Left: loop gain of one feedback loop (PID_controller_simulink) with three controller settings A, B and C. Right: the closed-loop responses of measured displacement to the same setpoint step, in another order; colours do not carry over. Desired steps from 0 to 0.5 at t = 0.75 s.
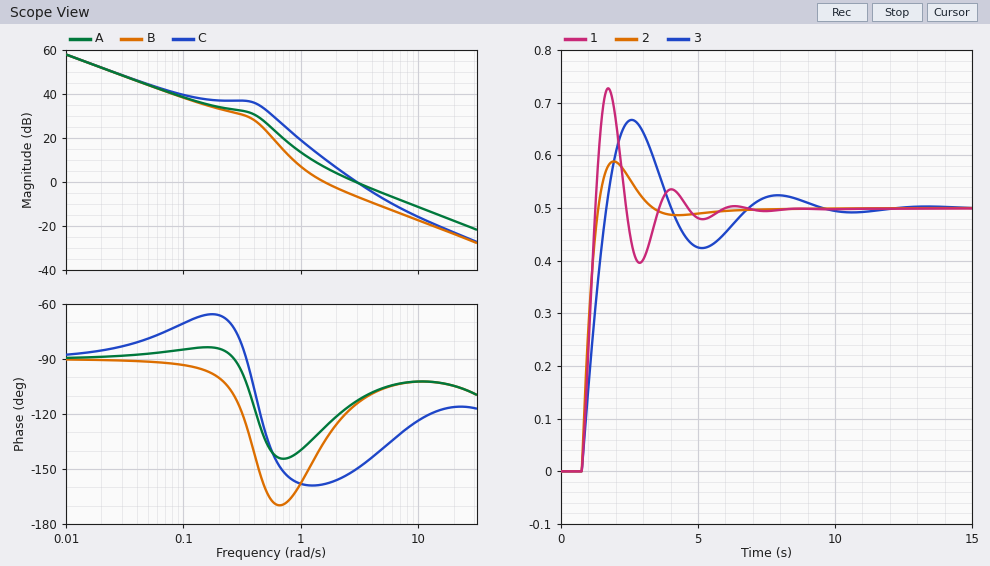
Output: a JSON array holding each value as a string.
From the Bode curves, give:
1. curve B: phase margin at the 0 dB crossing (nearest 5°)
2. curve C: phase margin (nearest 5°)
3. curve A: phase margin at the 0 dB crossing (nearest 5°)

["45°", "30°", "65°"]
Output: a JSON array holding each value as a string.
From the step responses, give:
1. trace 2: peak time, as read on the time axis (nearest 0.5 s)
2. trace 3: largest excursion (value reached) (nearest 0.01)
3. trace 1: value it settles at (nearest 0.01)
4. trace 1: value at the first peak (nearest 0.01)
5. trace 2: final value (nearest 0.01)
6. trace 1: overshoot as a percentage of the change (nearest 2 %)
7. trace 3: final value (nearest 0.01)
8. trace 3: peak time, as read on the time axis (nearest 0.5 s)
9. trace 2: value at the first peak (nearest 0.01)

["2.0 s", "0.67", "0.50", "0.73", "0.50", "46 %", "0.50", "2.5 s", "0.59"]
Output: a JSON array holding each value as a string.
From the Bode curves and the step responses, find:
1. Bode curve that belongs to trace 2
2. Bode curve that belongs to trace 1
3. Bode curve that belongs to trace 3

["A", "C", "B"]
